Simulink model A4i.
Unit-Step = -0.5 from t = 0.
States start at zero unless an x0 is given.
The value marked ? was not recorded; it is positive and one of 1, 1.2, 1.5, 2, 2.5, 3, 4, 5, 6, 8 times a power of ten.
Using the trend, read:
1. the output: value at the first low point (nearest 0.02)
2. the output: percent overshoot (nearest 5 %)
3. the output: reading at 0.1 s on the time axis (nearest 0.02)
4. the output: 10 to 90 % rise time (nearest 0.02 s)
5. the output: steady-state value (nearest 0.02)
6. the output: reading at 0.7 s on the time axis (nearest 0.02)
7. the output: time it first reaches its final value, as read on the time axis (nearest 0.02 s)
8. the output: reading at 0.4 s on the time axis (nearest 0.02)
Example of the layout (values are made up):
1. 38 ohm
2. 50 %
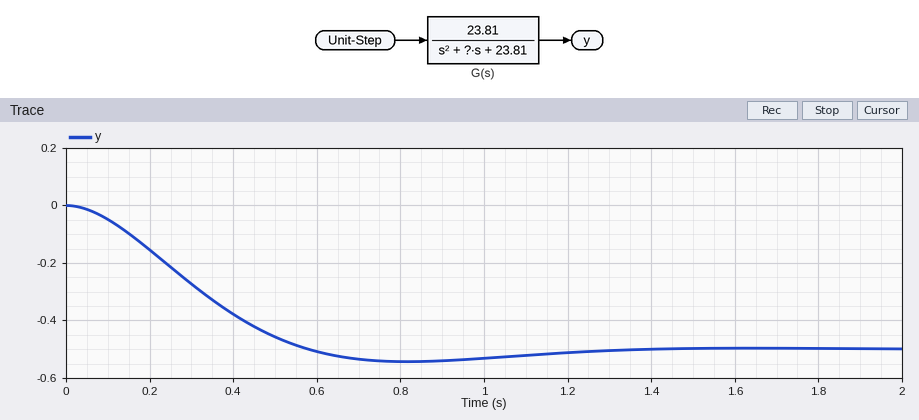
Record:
1. -0.54
2. 10 %
3. -0.04
4. 0.38 s
5. -0.50
6. -0.54
7. 0.58 s
8. -0.38
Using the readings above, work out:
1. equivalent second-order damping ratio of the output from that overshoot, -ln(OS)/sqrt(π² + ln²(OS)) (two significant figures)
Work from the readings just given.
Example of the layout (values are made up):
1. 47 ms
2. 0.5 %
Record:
1. 0.59
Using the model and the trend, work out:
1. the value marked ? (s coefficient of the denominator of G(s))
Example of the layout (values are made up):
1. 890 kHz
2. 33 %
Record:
1. 6
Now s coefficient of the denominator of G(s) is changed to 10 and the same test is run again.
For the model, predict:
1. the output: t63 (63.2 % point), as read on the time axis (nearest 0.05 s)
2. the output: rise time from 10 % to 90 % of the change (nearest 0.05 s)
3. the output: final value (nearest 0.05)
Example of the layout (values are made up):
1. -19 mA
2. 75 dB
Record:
1. 0.45 s
2. 0.70 s
3. -0.50
